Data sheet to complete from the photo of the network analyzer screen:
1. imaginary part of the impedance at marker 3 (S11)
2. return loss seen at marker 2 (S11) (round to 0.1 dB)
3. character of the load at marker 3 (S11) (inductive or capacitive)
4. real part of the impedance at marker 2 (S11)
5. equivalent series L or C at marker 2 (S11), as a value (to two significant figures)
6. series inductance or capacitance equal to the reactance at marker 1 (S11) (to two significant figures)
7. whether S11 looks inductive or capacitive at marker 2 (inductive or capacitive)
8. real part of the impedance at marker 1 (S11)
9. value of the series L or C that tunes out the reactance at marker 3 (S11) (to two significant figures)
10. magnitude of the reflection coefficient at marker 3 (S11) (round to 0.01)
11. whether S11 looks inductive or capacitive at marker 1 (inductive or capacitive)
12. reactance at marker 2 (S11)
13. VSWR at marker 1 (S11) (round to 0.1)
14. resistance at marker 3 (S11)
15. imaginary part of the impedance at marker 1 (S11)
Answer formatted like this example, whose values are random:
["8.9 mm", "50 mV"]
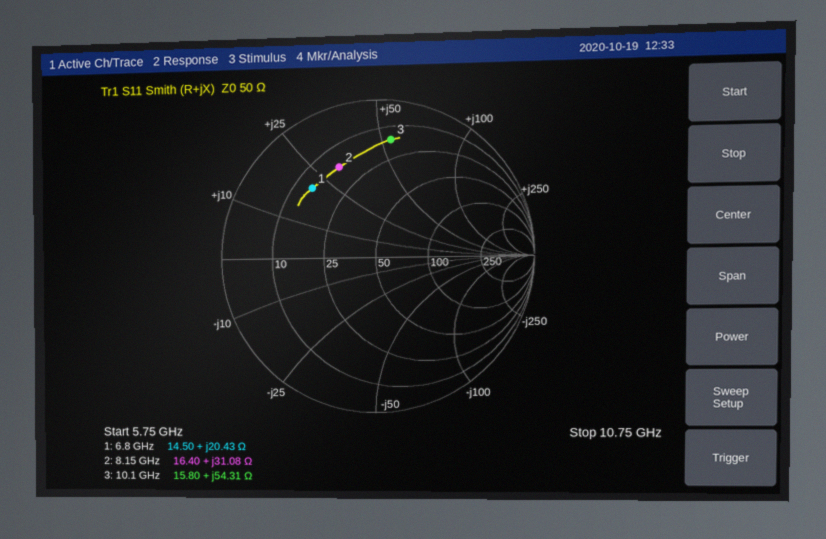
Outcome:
["+54.31 Ω", "4.1 dB", "inductive", "16.40 Ω", "610 pH", "480 pH", "inductive", "14.50 Ω", "290 fF", "0.75", "inductive", "+31.08 Ω", "4.1", "15.80 Ω", "+20.43 Ω"]
